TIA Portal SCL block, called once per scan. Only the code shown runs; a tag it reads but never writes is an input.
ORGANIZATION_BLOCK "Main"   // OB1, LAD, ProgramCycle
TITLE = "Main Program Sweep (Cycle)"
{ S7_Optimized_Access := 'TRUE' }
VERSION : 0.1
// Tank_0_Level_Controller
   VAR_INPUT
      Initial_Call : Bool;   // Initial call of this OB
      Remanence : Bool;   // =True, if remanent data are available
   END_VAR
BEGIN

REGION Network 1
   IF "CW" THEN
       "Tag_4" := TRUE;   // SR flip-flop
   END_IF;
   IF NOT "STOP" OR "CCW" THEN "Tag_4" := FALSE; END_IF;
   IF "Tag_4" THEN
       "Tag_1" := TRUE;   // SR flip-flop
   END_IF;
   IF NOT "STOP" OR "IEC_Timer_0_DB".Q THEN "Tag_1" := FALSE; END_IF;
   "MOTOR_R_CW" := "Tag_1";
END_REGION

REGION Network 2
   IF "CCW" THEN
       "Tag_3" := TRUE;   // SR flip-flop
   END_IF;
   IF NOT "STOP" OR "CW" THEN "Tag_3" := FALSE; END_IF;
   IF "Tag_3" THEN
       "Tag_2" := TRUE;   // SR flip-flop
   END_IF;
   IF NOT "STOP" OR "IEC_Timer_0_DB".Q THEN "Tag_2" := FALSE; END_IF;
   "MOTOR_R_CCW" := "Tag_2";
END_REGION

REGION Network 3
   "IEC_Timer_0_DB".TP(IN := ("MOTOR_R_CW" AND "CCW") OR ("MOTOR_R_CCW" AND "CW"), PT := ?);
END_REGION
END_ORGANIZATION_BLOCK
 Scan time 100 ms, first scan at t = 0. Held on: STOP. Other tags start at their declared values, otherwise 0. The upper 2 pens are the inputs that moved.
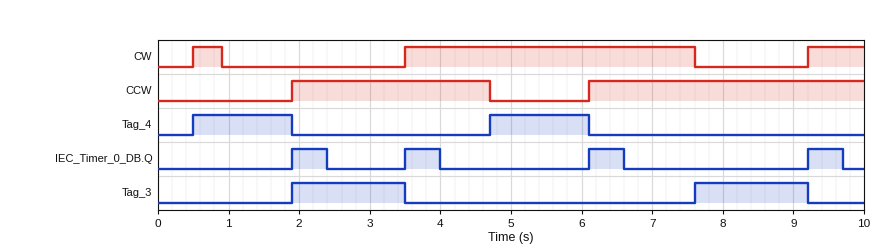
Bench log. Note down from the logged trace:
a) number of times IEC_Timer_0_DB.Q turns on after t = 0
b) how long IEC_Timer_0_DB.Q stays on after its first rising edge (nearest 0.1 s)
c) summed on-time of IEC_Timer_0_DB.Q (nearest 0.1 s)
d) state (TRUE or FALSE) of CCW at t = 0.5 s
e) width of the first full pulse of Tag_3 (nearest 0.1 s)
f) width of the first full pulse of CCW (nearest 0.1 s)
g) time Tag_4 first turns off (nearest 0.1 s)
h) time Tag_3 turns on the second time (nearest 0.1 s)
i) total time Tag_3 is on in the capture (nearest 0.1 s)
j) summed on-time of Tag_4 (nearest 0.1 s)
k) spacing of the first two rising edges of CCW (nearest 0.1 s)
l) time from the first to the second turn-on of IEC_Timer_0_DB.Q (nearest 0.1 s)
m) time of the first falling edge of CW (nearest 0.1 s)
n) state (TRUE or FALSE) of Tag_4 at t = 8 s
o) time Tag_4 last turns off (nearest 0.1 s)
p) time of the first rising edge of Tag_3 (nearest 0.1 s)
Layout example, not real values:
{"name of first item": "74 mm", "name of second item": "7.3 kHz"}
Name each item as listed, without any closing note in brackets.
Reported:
{"number of times IEC_Timer_0_DB.Q turns on after t = 0": "4", "how long IEC_Timer_0_DB.Q stays on after its first rising edge": "0.5 s", "summed on-time of IEC_Timer_0_DB.Q": "2.0 s", "state (TRUE or FALSE) of CCW at t = 0.5 s": "FALSE", "width of the first full pulse of Tag_3": "1.6 s", "width of the first full pulse of CCW": "2.8 s", "time Tag_4 first turns off": "1.9 s", "time Tag_3 turns on the second time": "7.6 s", "total time Tag_3 is on in the capture": "3.2 s", "summed on-time of Tag_4": "2.8 s", "spacing of the first two rising edges of CCW": "4.2 s", "time from the first to the second turn-on of IEC_Timer_0_DB.Q": "1.6 s", "time of the first falling edge of CW": "0.9 s", "state (TRUE or FALSE) of Tag_4 at t = 8 s": "FALSE", "time Tag_4 last turns off": "6.1 s", "time of the first rising edge of Tag_3": "1.9 s"}
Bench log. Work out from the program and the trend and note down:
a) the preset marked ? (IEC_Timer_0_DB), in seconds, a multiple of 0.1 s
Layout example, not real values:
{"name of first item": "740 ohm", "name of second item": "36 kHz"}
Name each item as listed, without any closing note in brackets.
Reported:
{"the preset marked ? (IEC_Timer_0_DB), in seconds, a multiple of 0.1 s": "0.5 s"}
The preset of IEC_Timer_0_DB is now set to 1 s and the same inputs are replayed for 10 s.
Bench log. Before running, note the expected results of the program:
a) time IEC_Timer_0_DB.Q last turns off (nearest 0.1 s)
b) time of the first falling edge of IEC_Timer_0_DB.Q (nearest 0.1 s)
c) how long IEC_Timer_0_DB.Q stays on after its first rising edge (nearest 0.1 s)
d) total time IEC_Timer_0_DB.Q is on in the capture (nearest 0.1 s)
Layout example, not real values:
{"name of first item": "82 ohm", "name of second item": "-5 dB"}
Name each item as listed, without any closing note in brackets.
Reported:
{"time IEC_Timer_0_DB.Q last turns off": "7.1 s", "time of the first falling edge of IEC_Timer_0_DB.Q": "2.9 s", "how long IEC_Timer_0_DB.Q stays on after its first rising edge": "1.0 s", "total time IEC_Timer_0_DB.Q is on in the capture": "3.8 s"}
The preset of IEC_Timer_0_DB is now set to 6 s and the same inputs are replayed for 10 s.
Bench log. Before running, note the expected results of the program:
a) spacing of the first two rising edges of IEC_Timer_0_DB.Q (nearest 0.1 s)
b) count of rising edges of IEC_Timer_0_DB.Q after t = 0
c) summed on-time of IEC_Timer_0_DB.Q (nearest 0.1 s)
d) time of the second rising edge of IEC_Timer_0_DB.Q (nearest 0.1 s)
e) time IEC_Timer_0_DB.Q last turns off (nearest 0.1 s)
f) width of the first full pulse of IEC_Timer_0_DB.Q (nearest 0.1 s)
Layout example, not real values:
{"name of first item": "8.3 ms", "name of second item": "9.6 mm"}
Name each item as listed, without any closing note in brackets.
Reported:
{"spacing of the first two rising edges of IEC_Timer_0_DB.Q": "7.3 s", "count of rising edges of IEC_Timer_0_DB.Q after t = 0": "2", "summed on-time of IEC_Timer_0_DB.Q": "6.8 s", "time of the second rising edge of IEC_Timer_0_DB.Q": "9.2 s", "time IEC_Timer_0_DB.Q last turns off": "7.9 s", "width of the first full pulse of IEC_Timer_0_DB.Q": "6.0 s"}
